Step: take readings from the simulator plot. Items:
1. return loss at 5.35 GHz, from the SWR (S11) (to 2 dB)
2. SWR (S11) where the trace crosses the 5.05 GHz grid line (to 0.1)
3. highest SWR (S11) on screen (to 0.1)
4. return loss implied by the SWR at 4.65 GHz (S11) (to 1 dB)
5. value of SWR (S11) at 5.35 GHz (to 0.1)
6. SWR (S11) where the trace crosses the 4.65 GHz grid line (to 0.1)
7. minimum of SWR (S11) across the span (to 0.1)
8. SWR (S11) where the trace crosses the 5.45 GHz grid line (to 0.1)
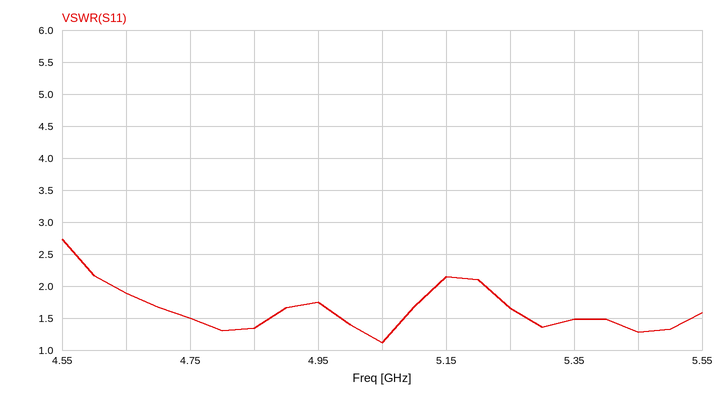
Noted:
14 dB
1.1
2.7
10 dB
1.5
1.9
1.1
1.3
